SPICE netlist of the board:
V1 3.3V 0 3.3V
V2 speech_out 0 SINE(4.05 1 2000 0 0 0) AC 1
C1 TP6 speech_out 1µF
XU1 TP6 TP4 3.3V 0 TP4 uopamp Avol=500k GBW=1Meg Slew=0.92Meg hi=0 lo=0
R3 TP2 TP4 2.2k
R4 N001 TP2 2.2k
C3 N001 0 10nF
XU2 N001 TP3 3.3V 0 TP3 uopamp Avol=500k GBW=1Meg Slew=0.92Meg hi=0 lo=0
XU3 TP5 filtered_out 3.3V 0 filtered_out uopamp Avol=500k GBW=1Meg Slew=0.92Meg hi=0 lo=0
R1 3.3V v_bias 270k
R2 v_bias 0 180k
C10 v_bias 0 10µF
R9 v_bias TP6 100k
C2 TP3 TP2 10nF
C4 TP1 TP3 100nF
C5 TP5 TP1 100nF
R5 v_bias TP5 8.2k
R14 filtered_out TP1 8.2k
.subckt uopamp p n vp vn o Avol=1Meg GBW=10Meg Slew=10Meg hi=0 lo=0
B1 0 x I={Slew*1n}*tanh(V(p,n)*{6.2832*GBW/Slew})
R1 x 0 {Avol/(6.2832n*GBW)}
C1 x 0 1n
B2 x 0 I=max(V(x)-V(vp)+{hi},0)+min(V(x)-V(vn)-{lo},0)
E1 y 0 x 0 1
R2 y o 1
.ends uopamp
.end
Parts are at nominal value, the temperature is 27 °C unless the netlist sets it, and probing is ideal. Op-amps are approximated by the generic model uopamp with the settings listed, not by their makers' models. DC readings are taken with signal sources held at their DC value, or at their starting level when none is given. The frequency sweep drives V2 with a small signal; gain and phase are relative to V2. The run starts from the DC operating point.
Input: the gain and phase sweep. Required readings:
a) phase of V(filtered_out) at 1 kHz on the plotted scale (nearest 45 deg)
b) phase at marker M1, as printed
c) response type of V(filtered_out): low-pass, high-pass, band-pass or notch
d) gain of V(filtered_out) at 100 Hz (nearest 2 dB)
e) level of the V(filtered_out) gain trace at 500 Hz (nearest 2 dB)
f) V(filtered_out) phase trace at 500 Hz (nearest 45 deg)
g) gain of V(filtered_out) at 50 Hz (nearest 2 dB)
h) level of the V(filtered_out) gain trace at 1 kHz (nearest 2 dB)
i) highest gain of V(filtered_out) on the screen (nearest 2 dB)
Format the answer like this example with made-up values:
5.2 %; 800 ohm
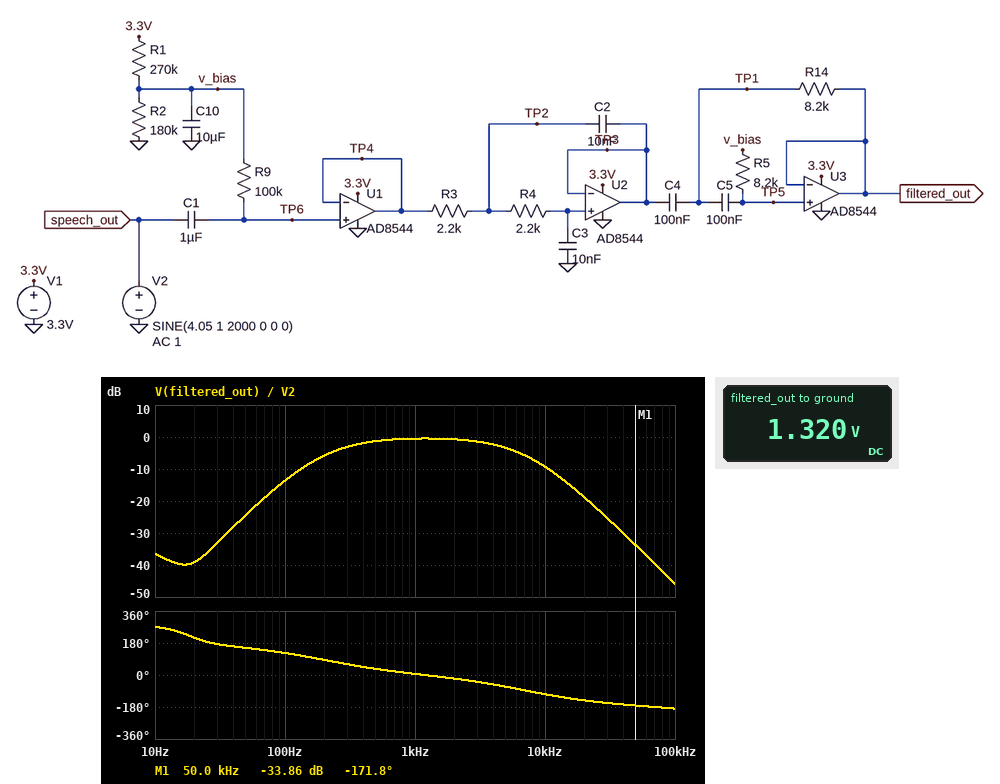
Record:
0 deg; -171.8 deg; band-pass; -14 dB; -2 dB; 45 deg; -24 dB; 0 dB; 0 dB
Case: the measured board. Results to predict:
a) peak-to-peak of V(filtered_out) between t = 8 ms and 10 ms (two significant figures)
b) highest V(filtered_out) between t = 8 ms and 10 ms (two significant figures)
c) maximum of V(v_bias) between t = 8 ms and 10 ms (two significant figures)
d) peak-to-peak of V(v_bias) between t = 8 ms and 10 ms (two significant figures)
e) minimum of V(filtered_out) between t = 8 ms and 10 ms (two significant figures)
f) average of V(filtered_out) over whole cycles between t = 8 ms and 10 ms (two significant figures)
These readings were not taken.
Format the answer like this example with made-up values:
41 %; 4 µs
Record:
1.8 V; 2.2 V; 1.3 V; 1.9 mV; 400 mV; 1.3 V
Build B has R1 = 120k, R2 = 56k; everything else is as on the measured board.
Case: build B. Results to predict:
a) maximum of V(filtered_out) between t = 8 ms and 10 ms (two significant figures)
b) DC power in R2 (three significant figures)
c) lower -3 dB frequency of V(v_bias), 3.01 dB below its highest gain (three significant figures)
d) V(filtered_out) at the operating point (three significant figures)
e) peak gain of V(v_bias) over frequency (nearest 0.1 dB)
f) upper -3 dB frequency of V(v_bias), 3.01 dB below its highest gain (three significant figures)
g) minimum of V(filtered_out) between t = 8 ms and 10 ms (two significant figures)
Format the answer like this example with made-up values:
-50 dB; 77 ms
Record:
2.0 V; 19.7 µW; 272 mHz; 1.05 V; -22.7 dB; 2.43 Hz; 130 mV
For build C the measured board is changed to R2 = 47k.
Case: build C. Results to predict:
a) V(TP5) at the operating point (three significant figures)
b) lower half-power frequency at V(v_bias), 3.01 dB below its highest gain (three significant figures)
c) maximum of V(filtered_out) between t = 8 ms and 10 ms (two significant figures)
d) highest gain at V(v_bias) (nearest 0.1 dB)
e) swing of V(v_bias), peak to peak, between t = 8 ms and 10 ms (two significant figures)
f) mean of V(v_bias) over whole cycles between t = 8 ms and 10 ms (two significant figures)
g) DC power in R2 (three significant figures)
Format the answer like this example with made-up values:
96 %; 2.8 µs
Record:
489 mV; 262 mHz; 1.3 V; -22.6 dB; 1.6 mV; 490 mV; 5.09 µW
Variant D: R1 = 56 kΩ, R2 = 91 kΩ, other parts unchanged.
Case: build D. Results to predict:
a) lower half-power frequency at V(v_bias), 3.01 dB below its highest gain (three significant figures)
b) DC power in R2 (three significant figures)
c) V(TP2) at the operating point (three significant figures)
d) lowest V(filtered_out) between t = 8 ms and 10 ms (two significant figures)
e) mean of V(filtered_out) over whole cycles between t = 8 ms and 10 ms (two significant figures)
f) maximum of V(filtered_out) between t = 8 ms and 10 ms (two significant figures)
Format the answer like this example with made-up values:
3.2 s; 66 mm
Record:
292 mHz; 45.9 µW; 2.04 V; 1.1 V; 2.0 V; 3.0 V
